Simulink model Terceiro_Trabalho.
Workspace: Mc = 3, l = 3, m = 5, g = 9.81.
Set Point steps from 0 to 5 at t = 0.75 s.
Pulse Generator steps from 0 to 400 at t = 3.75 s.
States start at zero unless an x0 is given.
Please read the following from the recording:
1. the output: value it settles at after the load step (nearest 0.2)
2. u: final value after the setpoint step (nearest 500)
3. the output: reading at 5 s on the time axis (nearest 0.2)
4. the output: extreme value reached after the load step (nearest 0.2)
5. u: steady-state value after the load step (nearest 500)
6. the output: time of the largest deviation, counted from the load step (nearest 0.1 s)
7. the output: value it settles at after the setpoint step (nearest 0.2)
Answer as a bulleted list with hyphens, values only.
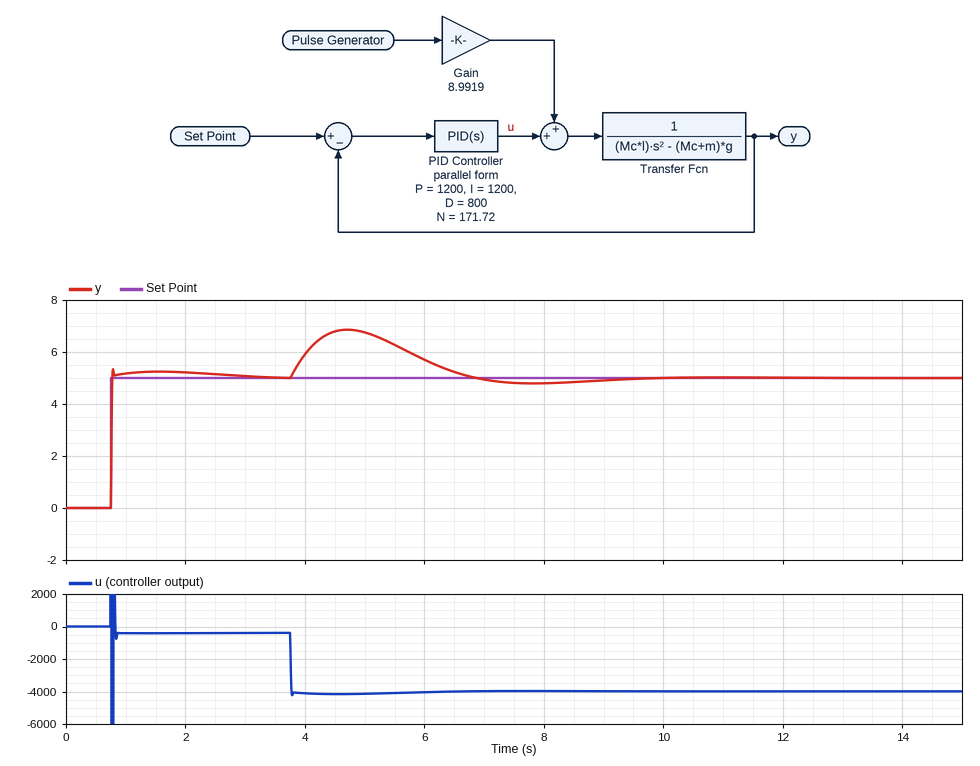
- 5.0
- -500
- 6.8
- 6.8
- -4000
- 1.0 s
- 5.0
